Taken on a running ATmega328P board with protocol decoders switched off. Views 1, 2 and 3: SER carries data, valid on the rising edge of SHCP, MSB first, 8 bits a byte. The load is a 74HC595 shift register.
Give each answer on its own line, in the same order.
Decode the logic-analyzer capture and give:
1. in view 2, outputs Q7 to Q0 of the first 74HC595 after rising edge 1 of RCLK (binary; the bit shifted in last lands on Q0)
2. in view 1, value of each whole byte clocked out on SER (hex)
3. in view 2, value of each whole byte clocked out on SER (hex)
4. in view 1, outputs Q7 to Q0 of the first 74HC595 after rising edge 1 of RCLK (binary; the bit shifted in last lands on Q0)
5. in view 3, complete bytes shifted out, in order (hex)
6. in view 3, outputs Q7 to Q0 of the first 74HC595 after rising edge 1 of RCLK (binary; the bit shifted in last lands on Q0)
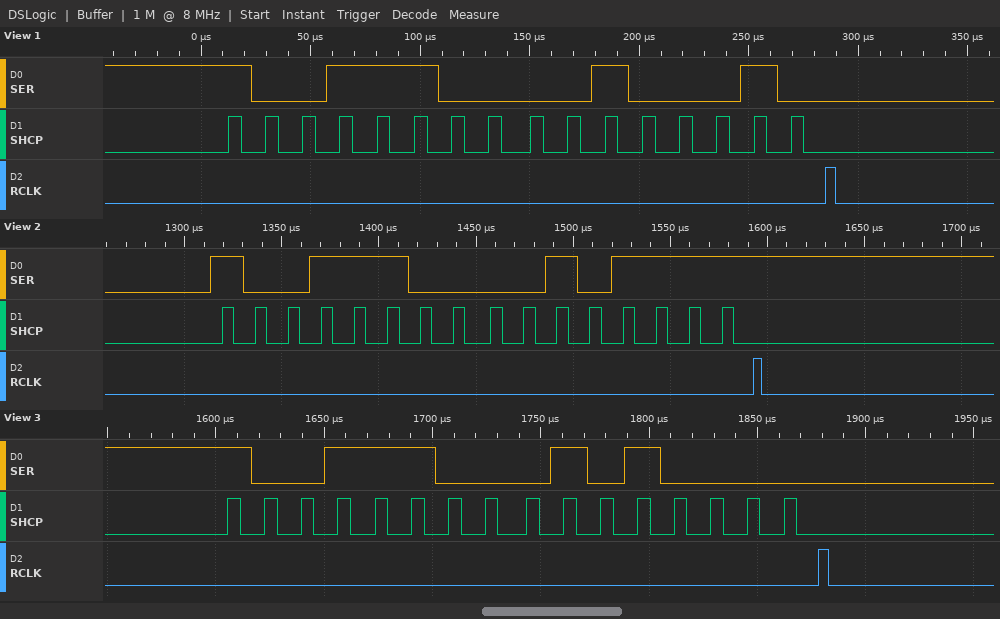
00101111
9C 22
9C 2F
00100010
0x9C 0x50
01010000
